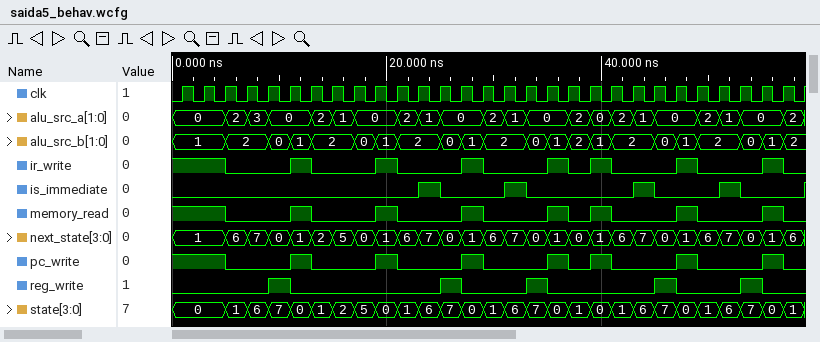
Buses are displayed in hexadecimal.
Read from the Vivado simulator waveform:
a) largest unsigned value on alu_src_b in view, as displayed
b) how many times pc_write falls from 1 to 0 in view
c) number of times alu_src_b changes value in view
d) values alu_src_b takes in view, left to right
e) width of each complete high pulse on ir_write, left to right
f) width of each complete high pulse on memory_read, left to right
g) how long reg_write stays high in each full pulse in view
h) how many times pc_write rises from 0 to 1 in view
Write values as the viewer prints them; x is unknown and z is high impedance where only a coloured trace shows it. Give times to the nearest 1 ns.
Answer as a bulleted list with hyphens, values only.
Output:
- 2
- 8
- 21
- 1, 2, 0, 1, 2, 0, 1, 2, 0, 1, 2, 0, 1, 2, 1, 2, 0, 1, 2, 0, 1, 2
- 2 ns, 2 ns, 2 ns, 2 ns, 2 ns, 2 ns, 2 ns
- 2 ns, 2 ns, 2 ns, 2 ns, 2 ns, 2 ns, 2 ns
- 2 ns, 2 ns, 2 ns, 2 ns, 2 ns
- 7
